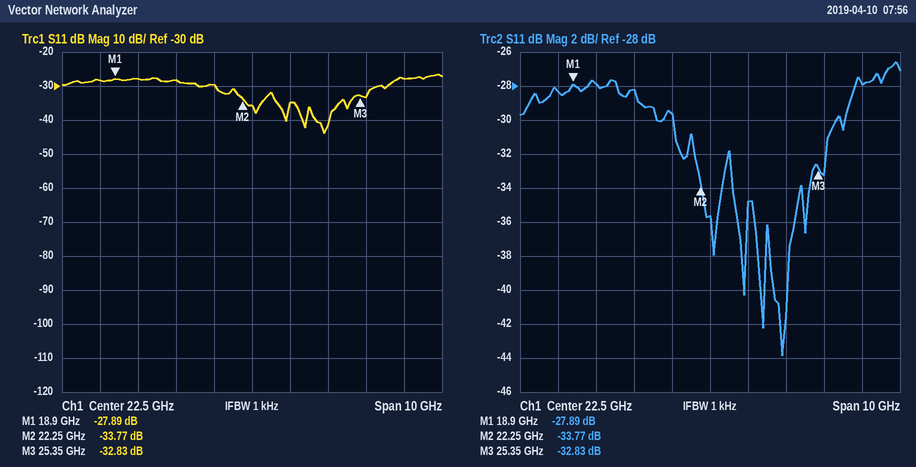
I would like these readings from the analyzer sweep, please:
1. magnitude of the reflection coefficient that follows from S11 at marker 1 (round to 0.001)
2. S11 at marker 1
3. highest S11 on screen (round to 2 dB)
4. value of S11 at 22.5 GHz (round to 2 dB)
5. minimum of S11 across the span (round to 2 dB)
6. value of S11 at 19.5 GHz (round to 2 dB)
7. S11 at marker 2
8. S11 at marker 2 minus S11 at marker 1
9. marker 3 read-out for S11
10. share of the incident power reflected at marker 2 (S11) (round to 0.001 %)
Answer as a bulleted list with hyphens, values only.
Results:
- 0.040
- -27.89 dB
- -26 dB
- -36 dB
- -44 dB
- -28 dB
- -33.77 dB
- -5.88 dB
- -32.83 dB
- 0.042 %
